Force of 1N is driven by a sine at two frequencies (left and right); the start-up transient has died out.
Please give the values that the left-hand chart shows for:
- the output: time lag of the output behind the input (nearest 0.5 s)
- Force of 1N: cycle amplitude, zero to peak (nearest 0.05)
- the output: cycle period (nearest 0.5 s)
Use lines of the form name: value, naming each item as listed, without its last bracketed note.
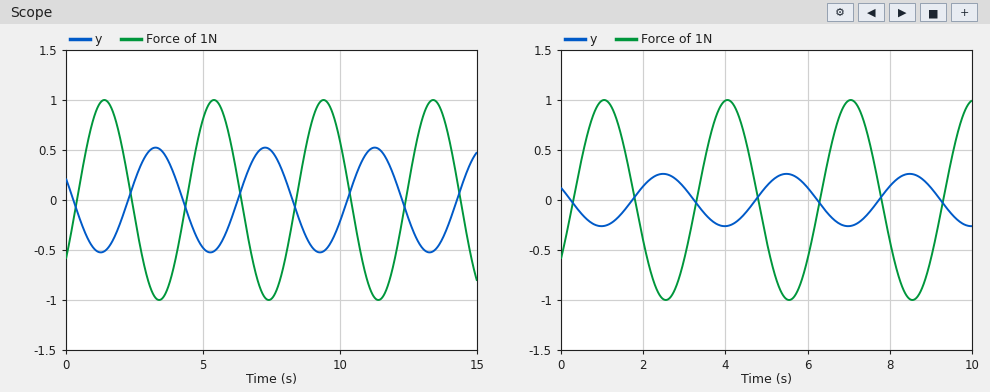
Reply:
the output: time lag of the output behind the input: 2.0 s
Force of 1N: cycle amplitude, zero to peak: 1.00
the output: cycle period: 4.0 s
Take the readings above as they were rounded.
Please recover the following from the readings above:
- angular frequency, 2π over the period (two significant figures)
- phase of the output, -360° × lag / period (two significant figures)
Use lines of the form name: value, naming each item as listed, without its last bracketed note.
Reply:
angular frequency, 2π over the period: 1.6 rad/s
phase of the output, -360° × lag / period: -180°
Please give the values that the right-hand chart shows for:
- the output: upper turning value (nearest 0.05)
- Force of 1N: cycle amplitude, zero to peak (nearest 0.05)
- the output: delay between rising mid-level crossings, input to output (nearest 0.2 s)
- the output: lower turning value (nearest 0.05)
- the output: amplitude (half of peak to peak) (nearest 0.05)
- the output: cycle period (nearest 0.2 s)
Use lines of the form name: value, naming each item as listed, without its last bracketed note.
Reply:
the output: upper turning value: 0.25
Force of 1N: cycle amplitude, zero to peak: 1.00
the output: delay between rising mid-level crossings, input to output: 1.4 s
the output: lower turning value: -0.25
the output: amplitude (half of peak to peak): 0.25
the output: cycle period: 3.0 s
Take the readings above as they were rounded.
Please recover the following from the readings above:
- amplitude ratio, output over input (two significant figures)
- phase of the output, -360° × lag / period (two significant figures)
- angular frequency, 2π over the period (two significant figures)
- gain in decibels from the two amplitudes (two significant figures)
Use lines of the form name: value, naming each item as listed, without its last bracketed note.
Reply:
amplitude ratio, output over input: 0.25
phase of the output, -360° × lag / period: -170°
angular frequency, 2π over the period: 2.1 rad/s
gain in decibels from the two amplitudes: -12 dB
